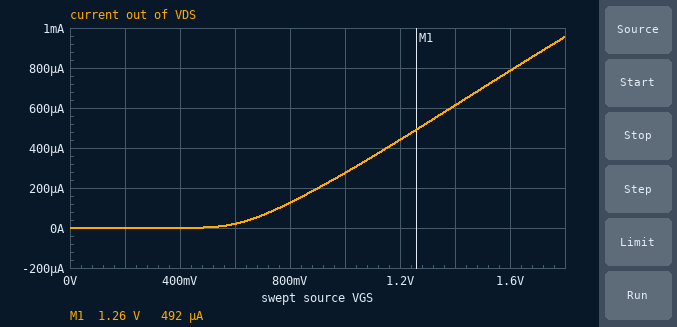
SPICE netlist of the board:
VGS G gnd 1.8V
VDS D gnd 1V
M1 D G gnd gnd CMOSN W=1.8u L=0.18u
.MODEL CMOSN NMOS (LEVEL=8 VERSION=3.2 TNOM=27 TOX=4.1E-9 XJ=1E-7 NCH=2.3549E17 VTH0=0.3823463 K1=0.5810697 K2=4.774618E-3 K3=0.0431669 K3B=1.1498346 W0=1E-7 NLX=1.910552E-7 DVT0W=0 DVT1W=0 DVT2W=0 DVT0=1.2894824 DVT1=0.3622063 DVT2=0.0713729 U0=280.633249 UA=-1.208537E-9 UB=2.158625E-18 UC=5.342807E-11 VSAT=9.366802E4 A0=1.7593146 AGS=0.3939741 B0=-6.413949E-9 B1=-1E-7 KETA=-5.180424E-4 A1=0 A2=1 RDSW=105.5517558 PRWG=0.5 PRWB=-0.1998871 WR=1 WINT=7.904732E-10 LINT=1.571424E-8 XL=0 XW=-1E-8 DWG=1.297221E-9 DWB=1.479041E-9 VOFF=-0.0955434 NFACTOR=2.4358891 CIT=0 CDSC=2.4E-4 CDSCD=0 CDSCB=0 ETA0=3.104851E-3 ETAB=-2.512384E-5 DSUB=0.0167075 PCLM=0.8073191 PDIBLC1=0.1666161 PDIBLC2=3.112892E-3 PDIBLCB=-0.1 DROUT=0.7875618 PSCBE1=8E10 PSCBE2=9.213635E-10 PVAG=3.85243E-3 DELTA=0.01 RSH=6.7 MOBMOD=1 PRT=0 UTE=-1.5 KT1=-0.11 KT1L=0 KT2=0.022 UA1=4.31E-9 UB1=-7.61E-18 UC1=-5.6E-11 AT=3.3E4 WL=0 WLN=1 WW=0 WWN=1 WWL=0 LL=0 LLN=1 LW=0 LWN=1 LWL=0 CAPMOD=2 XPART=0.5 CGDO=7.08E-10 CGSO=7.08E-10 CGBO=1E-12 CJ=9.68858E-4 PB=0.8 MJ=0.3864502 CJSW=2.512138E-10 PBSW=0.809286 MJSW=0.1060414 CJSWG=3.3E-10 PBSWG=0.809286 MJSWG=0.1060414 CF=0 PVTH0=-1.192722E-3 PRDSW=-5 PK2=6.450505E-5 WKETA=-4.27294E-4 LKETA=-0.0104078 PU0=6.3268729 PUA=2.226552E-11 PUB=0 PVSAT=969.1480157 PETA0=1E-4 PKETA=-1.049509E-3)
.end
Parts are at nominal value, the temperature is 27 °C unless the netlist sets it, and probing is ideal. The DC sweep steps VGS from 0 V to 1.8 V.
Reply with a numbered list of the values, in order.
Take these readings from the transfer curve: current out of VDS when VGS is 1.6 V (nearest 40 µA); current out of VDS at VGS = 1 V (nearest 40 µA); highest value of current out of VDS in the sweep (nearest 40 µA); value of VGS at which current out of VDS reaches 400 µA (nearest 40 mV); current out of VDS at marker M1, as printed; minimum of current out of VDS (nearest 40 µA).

1. 800 µA
2. 280 µA
3. 960 µA
4. 1.16 V
5. 492 µA
6. 0 A
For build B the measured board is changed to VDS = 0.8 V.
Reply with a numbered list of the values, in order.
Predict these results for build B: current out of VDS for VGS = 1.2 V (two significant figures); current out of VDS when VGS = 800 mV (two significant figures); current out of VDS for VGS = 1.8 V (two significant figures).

1. 430 µA
2. 120 µA
3. 930 µA
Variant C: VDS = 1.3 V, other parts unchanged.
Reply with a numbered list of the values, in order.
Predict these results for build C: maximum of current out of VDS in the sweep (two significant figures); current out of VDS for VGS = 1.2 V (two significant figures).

1. 980 µA
2. 450 µA
